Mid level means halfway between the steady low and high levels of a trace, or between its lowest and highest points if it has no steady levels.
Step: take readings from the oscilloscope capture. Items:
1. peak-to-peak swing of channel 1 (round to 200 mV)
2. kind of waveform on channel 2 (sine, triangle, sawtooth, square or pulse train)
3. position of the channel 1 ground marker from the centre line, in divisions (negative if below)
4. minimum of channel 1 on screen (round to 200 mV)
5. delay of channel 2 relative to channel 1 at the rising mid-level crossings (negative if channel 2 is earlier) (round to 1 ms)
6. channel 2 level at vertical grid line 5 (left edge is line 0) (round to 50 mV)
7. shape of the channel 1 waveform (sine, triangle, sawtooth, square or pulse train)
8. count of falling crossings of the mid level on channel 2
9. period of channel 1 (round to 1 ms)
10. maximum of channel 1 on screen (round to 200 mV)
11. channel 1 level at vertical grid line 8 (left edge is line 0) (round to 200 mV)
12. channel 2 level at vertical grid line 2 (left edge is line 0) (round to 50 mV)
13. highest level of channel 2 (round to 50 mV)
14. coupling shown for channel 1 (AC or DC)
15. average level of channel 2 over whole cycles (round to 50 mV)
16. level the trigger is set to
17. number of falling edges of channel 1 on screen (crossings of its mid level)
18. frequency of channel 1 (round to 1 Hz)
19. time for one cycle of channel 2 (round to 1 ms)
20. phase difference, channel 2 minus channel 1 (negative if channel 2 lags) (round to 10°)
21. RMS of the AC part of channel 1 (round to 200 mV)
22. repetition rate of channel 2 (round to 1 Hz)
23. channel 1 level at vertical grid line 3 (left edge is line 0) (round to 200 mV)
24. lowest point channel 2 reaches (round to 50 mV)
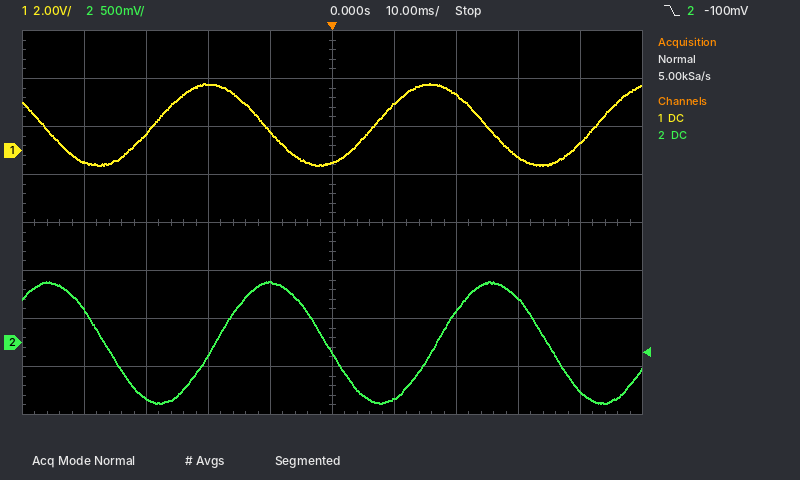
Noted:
3.4 V
sine
+1.5 div
-600 mV
+10 ms
-100 mV
sine
3
36 ms
2.8 V
-200 mV
-600 mV
650 mV
DC
0 mV
-100 mV
3
28 Hz
36 ms
-100°
1.2 V
28 Hz
2.8 V
-650 mV
